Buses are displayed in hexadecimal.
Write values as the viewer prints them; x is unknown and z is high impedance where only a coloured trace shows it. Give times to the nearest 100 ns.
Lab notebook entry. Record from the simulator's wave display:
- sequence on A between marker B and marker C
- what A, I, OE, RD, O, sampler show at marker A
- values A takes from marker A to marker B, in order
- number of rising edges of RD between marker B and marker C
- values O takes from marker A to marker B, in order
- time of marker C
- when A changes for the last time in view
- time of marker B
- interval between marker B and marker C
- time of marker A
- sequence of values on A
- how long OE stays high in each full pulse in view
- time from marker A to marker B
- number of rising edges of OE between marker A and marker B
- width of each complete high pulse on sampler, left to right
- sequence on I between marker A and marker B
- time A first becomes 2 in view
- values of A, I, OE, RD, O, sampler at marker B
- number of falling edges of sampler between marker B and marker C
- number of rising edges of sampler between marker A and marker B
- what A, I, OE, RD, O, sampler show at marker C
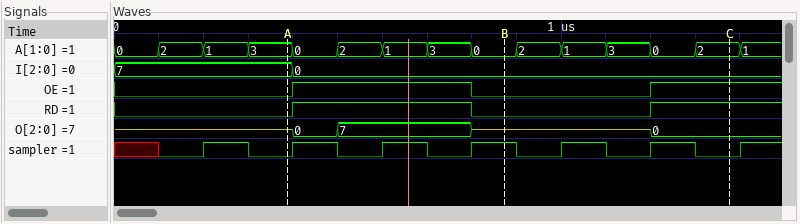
0, 2, 1, 3, 0, 2
A=3, I=7, OE=0, RD=0, O=z, sampler=0
3, 0, 2, 1, 3, 0
1
z, 0, 7, z
1400 ns
1400 ns
900 ns
500 ns
400 ns
0, 2, 1, 3, 0, 2, 1, 3, 0, 2, 1, 3, 0, 2, 1
400 ns
500 ns
1
100 ns, 100 ns, 100 ns, 100 ns, 100 ns, 100 ns
7, 0
100 ns
A=0, I=0, OE=0, RD=0, O=z, sampler=1
3
3
A=2, I=0, OE=1, RD=1, O=0, sampler=0
